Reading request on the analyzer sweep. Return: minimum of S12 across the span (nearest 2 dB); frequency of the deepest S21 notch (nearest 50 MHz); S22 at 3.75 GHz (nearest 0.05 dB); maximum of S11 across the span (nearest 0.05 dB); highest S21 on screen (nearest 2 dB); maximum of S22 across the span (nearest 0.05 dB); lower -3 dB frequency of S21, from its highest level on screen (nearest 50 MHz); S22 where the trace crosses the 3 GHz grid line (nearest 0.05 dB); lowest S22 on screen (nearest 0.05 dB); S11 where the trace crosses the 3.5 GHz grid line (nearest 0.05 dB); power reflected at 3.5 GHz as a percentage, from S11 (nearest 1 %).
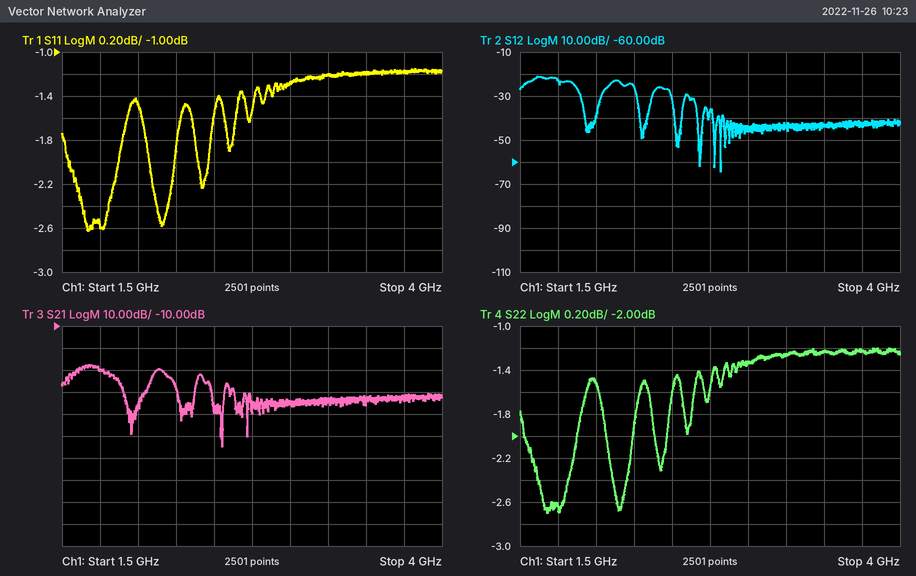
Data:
-64 dB
2.55 GHz
-1.20 dB
-1.15 dB
-28 dB
-1.20 dB
1.60 GHz
-1.35 dB
-2.70 dB
-1.20 dB
76 %
